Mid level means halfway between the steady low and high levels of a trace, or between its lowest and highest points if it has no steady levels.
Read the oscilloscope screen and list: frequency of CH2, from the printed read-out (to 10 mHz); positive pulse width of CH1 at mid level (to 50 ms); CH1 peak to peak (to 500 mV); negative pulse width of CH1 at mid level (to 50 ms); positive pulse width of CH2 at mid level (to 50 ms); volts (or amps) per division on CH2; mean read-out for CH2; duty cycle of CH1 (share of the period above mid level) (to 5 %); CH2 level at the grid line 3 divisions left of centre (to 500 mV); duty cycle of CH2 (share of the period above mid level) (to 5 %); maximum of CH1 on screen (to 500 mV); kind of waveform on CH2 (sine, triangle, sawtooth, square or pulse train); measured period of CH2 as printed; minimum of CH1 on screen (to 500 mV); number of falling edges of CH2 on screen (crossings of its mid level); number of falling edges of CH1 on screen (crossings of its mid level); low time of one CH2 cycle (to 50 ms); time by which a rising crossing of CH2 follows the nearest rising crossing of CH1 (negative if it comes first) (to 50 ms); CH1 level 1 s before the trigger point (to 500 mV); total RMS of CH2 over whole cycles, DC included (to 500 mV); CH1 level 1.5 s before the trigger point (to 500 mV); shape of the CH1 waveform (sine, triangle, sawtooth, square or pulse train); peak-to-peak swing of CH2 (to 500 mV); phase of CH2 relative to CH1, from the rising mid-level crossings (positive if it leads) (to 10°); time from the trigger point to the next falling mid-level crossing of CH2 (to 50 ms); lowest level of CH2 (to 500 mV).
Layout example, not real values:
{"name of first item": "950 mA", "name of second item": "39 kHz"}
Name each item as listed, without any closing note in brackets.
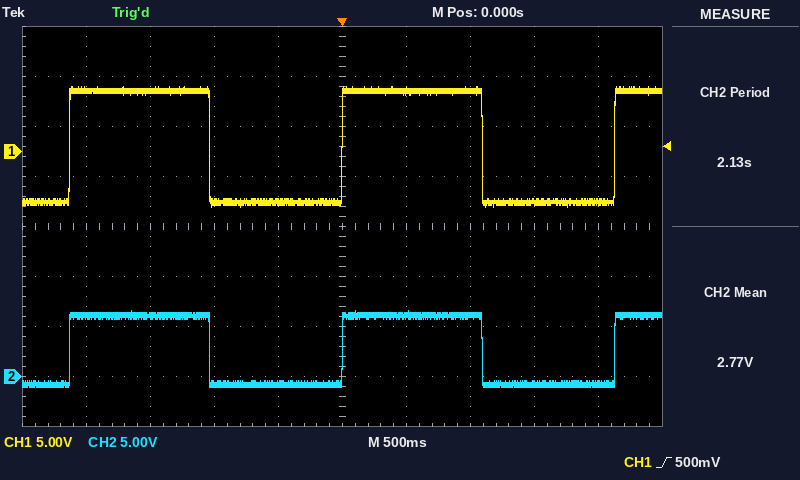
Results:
{"frequency of CH2, from the printed read-out": "470 mHz", "positive pulse width of CH1 at mid level": "1.10 s", "CH1 peak to peak": "12.0 V", "negative pulse width of CH1 at mid level": "1.05 s", "positive pulse width of CH2 at mid level": "1.10 s", "volts (or amps) per division on CH2": "5 V", "mean read-out for CH2": "2.77 V", "duty cycle of CH1 (share of the period above mid level)": "50 %", "CH2 level at the grid line 3 divisions left of centre": "6.0 V", "duty cycle of CH2 (share of the period above mid level)": "50 %", "maximum of CH1 on screen": "6.5 V", "kind of waveform on CH2": "square", "measured period of CH2 as printed": "2.13 s", "minimum of CH1 on screen": "-5.5 V", "number of falling edges of CH2 on screen": "2", "number of falling edges of CH1 on screen": "2", "low time of one CH2 cycle": "1.05 s", "time by which a rising crossing of CH2 follows the nearest rising crossing of CH1 (negative if it comes first)": "0 ms", "CH1 level 1 s before the trigger point": "-5.0 V", "total RMS of CH2 over whole cycles, DC included": "4.5 V", "CH1 level 1.5 s before the trigger point": "6.0 V", "shape of the CH1 waveform": "square", "peak-to-peak swing of CH2": "7.5 V", "phase of CH2 relative to CH1, from the rising mid-level crossings (positive if it leads)": "0°", "time from the trigger point to the next falling mid-level crossing of CH2": "1.10 s", "lowest level of CH2": "-1.0 V"}
